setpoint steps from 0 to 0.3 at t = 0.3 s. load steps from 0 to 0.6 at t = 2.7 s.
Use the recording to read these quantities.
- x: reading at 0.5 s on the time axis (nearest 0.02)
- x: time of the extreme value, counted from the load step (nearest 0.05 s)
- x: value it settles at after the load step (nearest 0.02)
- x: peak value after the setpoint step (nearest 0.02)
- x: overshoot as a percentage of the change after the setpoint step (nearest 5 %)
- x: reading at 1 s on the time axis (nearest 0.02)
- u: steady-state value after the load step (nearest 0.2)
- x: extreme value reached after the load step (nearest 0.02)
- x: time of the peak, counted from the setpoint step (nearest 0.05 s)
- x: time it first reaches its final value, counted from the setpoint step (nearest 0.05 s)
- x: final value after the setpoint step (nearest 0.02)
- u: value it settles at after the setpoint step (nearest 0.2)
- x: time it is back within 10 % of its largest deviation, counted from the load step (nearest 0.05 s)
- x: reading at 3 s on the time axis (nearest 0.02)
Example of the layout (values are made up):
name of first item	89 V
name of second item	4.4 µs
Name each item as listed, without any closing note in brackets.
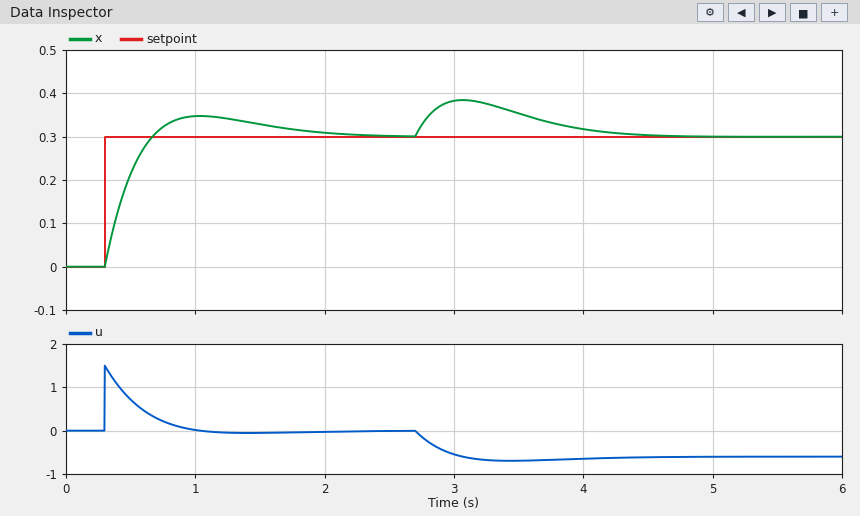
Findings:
x: reading at 0.5 s on the time axis	0.22
x: time of the extreme value, counted from the load step	0.35 s
x: value it settles at after the load step	0.30
x: peak value after the setpoint step	0.34
x: overshoot as a percentage of the change after the setpoint step	15 %
x: reading at 1 s on the time axis	0.34
u: steady-state value after the load step	-0.6
x: extreme value reached after the load step	0.38
x: time of the peak, counted from the setpoint step	0.75 s
x: time it first reaches its final value, counted from the setpoint step	0.35 s
x: final value after the setpoint step	0.30
u: value it settles at after the setpoint step	0.0
x: time it is back within 10 % of its largest deviation, counted from the load step	1.55 s
x: reading at 3 s on the time axis	0.38
